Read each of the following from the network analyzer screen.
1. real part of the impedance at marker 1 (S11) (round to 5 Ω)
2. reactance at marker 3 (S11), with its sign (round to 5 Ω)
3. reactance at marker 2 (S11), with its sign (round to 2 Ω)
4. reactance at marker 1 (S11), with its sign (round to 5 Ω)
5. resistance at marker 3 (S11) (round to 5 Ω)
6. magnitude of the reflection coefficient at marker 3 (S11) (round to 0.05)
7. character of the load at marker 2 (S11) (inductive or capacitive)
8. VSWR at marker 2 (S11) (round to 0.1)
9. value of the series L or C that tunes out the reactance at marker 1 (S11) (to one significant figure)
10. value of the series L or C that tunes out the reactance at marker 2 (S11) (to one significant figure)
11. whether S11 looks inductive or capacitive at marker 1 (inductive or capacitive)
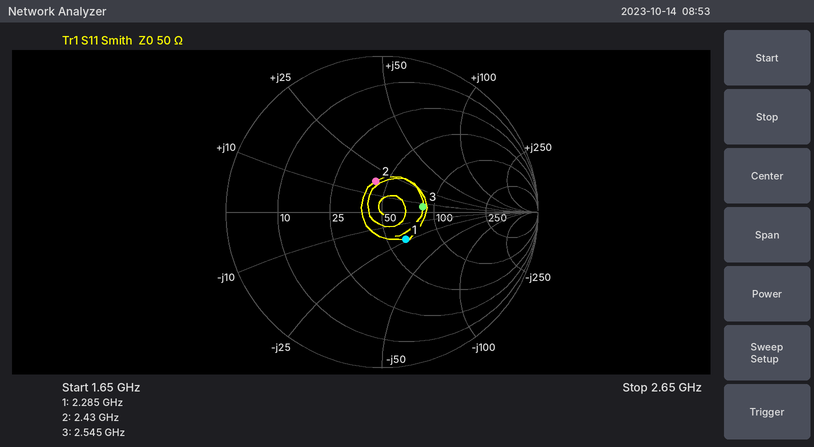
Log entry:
65 Ω
+5 Ω
+18 Ω
-25 Ω
85 Ω
0.25
inductive
1.5
2 nH
4 pF
capacitive
